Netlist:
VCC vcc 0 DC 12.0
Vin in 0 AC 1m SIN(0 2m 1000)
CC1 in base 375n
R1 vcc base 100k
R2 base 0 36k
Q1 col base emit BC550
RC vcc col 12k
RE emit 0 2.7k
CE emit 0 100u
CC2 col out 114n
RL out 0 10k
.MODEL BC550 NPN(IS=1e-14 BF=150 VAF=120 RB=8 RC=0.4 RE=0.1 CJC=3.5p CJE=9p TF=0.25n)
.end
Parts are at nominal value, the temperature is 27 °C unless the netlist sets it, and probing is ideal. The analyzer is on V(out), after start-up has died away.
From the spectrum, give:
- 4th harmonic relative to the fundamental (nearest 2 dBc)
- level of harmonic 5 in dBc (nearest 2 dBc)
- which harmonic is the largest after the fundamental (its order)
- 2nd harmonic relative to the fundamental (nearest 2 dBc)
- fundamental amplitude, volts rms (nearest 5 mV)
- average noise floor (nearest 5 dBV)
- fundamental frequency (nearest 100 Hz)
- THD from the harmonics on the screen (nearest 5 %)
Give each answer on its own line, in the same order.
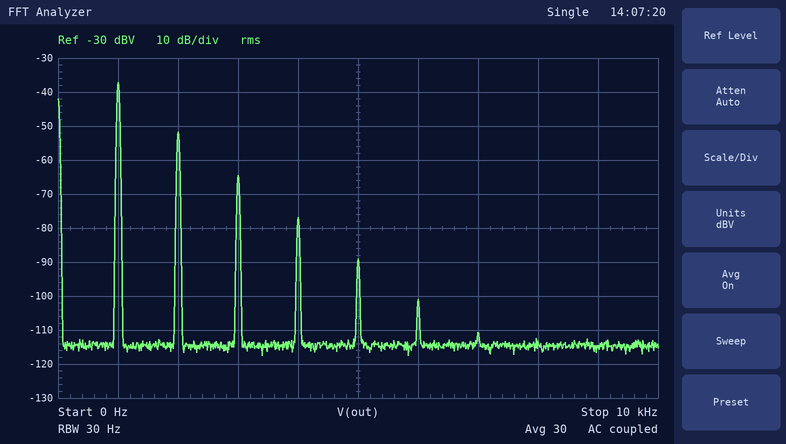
-40 dBc
-52 dBc
2
-14 dBc
15 mV
-115 dBV
1.0 kHz
20 %
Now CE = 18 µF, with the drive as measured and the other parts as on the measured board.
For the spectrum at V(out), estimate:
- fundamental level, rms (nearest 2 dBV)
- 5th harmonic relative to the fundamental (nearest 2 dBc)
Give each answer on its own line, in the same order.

-38 dBV
-54 dBc
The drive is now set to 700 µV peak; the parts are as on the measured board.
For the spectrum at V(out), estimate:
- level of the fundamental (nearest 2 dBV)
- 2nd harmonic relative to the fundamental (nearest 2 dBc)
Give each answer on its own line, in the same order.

-48 dBV
-24 dBc
